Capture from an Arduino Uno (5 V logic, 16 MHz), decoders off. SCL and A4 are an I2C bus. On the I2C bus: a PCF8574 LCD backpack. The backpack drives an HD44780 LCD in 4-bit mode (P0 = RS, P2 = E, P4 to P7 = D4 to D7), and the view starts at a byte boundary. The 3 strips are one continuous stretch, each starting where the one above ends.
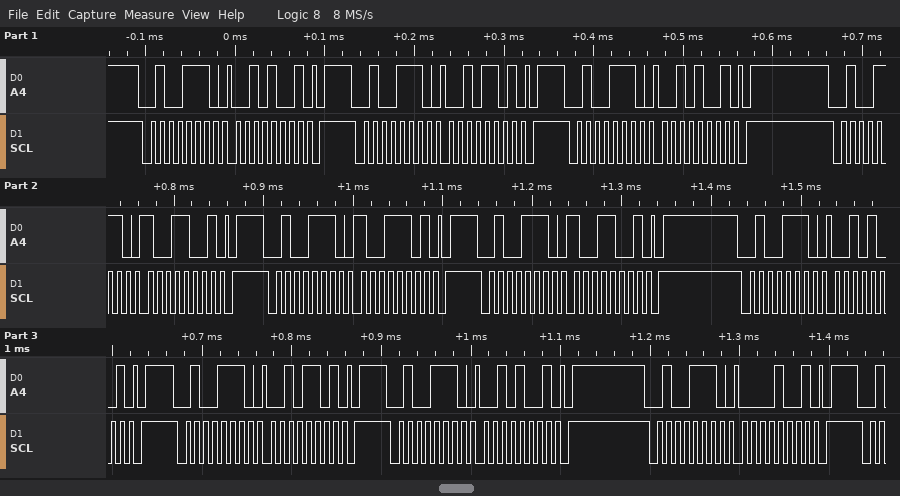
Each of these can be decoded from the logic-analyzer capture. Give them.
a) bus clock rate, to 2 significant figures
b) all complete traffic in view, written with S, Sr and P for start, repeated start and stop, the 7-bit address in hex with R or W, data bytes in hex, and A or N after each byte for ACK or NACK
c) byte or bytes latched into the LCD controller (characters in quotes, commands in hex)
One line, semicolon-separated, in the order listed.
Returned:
100 kHz; S 27W A 29 A P S 27W A 2D A P S 27W A 29 A P S 27W A 99 A P S 27W A 9D A P S 27W A 99 A P S 27W A 29 A P S 27W A 2D A P S 27W A 29 A P S 27W A 09 A P; ')'
